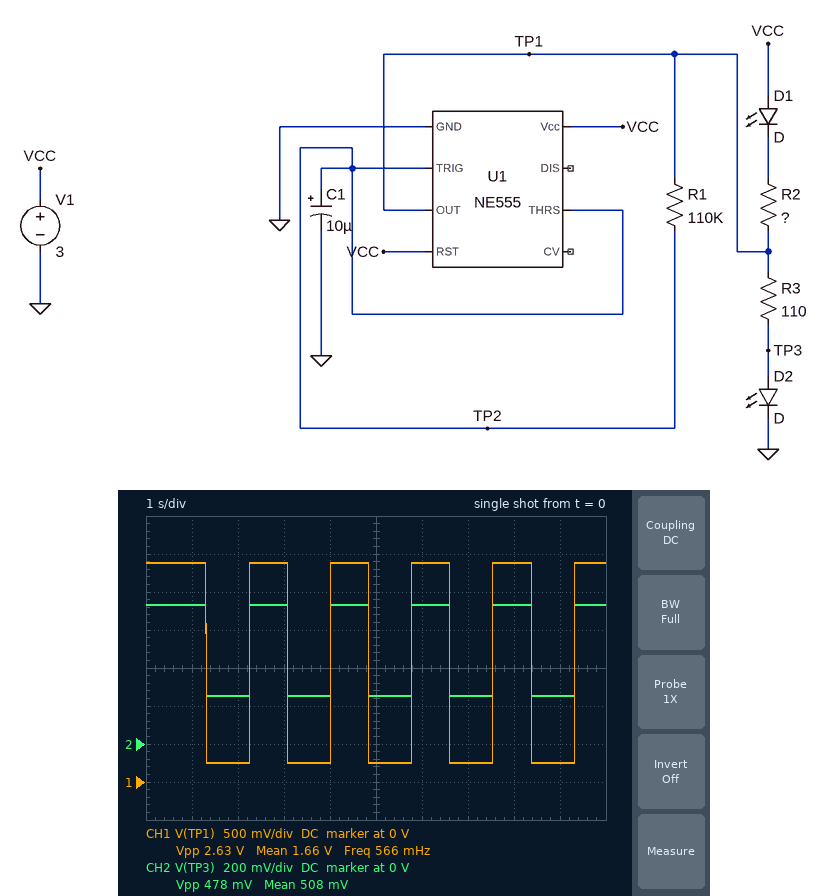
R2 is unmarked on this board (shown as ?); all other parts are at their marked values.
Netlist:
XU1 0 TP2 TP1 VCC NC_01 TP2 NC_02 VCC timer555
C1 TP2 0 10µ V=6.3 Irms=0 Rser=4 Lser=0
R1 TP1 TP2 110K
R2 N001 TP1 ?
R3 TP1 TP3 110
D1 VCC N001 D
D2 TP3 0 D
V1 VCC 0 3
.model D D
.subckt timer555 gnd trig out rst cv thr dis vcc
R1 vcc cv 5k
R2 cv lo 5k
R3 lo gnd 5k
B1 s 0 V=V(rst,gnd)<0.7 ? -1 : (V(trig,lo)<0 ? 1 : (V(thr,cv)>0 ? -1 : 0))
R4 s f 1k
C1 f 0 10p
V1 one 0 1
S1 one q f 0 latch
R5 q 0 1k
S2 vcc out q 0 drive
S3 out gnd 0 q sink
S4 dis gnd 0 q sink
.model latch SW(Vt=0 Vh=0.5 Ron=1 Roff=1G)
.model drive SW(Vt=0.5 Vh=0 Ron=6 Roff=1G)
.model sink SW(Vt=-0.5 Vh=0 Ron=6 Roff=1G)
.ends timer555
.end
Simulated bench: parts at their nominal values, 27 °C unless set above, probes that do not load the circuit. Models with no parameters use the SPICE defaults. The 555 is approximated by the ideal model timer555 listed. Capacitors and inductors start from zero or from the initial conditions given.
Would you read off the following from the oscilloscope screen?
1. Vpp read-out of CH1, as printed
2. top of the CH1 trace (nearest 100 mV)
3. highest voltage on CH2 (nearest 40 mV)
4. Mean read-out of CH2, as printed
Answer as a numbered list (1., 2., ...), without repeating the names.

1. 2.63 V
2. 2.9 V
3. 720 mV
4. 508 mV
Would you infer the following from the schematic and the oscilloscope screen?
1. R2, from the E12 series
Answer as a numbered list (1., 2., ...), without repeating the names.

1. 47 Ω
